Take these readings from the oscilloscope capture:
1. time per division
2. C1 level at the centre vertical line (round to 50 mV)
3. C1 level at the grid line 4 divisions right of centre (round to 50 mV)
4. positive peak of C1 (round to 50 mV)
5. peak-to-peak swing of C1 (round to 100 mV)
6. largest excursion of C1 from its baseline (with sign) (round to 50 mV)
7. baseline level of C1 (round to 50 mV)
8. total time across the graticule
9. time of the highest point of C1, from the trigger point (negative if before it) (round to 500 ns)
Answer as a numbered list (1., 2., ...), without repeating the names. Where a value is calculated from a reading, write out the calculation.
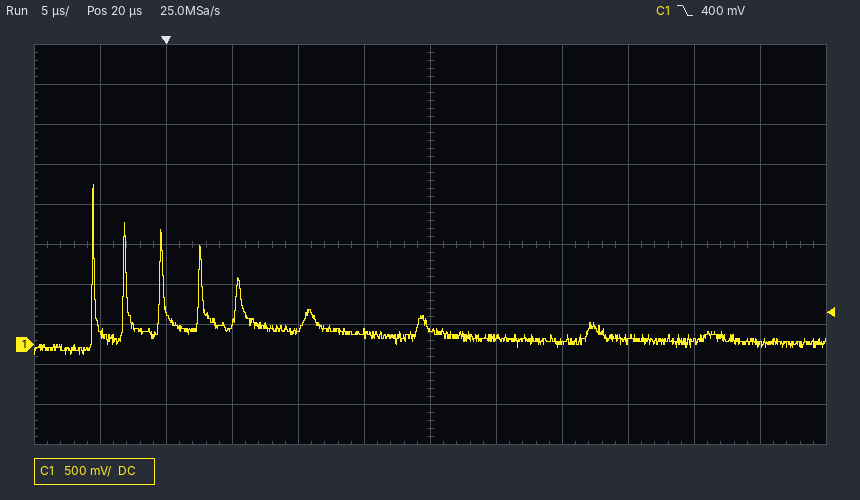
1. 5 µs
2. 200 mV
3. 50 mV
4. 2.00 V
5. 2.10 V
6. 2.00 V − (100 mV) = +1.90 V
7. 100 mV
8. 60 µs
9. -5.5 µs
